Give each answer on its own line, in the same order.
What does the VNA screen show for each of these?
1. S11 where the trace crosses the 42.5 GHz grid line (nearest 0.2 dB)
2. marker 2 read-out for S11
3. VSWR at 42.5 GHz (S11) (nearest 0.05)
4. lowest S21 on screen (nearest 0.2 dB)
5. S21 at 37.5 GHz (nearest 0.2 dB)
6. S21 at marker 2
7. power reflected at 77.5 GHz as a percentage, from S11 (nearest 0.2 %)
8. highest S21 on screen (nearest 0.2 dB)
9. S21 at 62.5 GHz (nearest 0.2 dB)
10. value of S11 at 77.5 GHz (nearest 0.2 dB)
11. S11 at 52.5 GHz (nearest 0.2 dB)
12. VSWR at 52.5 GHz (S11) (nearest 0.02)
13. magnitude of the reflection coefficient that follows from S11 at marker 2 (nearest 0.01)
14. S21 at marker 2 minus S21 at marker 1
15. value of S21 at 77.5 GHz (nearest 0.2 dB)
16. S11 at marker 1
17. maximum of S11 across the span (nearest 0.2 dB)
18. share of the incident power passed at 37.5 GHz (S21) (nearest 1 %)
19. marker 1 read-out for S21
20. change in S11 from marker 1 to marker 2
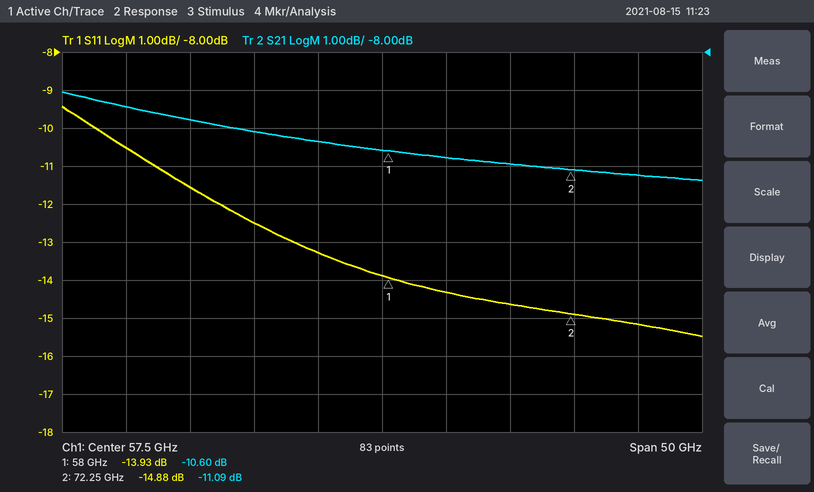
-11.6 dB
-14.88 dB
1.70
-11.4 dB
-9.4 dB
-11.09 dB
3.0 %
-9.0 dB
-10.8 dB
-15.2 dB
-13.2 dB
1.56
0.18
-0.49 dB
-11.2 dB
-13.93 dB
-9.4 dB
11 %
-10.60 dB
-0.95 dB
